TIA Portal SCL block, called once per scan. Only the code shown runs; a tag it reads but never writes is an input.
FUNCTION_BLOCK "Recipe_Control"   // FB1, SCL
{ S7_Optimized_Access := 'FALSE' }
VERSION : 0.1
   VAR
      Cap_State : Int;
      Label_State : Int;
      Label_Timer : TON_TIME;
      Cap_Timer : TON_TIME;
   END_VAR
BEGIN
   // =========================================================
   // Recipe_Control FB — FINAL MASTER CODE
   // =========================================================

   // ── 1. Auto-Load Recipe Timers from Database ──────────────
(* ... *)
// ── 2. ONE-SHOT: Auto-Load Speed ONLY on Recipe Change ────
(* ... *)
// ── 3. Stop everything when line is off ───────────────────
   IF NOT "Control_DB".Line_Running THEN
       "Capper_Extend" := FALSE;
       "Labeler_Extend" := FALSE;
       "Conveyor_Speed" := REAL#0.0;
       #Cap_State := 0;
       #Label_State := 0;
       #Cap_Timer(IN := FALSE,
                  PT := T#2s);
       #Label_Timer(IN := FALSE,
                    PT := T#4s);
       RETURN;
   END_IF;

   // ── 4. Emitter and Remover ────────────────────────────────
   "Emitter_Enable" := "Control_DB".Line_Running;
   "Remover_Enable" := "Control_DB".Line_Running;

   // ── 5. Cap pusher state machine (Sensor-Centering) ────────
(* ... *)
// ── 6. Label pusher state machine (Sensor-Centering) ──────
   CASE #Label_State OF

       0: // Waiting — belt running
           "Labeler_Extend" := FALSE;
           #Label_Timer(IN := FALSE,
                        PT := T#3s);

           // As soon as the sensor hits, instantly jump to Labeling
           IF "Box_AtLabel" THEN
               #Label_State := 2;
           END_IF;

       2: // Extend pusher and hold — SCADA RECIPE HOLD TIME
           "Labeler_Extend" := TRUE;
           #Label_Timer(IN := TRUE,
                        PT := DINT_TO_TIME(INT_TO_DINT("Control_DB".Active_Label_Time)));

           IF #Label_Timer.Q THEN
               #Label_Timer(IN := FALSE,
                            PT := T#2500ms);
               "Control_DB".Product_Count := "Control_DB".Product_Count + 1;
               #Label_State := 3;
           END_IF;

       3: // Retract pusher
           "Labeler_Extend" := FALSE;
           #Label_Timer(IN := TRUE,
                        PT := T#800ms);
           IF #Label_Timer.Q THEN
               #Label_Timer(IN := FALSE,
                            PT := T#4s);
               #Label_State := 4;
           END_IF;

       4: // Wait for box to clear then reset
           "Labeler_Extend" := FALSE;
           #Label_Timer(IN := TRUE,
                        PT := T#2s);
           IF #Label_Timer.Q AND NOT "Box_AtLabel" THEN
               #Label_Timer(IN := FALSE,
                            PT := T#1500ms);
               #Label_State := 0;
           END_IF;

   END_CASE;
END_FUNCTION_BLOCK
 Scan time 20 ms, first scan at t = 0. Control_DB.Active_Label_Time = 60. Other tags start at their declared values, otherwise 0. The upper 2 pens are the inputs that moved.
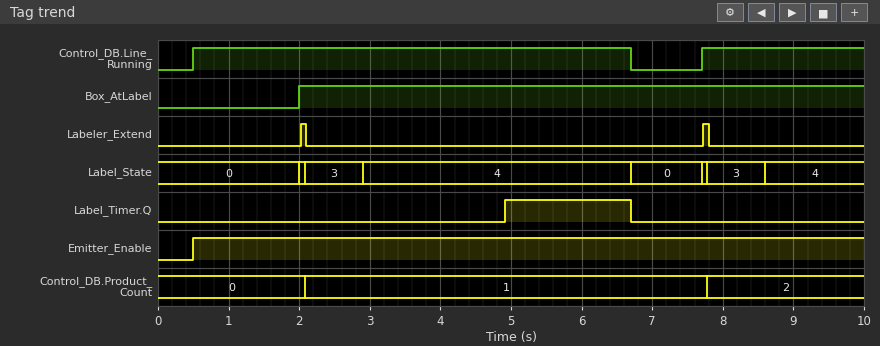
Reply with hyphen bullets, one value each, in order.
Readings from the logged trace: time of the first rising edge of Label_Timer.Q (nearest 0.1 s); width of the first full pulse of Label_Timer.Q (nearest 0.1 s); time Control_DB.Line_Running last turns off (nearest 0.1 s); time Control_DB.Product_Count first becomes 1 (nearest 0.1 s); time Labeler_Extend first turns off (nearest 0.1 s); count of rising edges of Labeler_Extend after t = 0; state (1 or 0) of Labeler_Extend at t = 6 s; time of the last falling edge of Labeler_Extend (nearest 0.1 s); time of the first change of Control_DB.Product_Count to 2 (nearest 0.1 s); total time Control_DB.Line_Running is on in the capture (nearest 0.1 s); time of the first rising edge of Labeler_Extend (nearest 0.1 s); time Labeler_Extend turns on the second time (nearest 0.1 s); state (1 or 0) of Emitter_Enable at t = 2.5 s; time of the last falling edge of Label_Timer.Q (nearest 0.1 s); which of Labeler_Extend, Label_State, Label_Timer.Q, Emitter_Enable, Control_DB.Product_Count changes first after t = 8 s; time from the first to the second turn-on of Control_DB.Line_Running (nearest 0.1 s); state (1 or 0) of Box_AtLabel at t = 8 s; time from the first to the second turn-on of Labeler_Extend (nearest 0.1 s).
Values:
- 4.9 s
- 1.8 s
- 6.7 s
- 2.1 s
- 2.1 s
- 2
- 0
- 7.8 s
- 7.8 s
- 8.5 s
- 2.0 s
- 7.7 s
- 1
- 6.7 s
- Label_State
- 7.2 s
- 1
- 5.7 s
